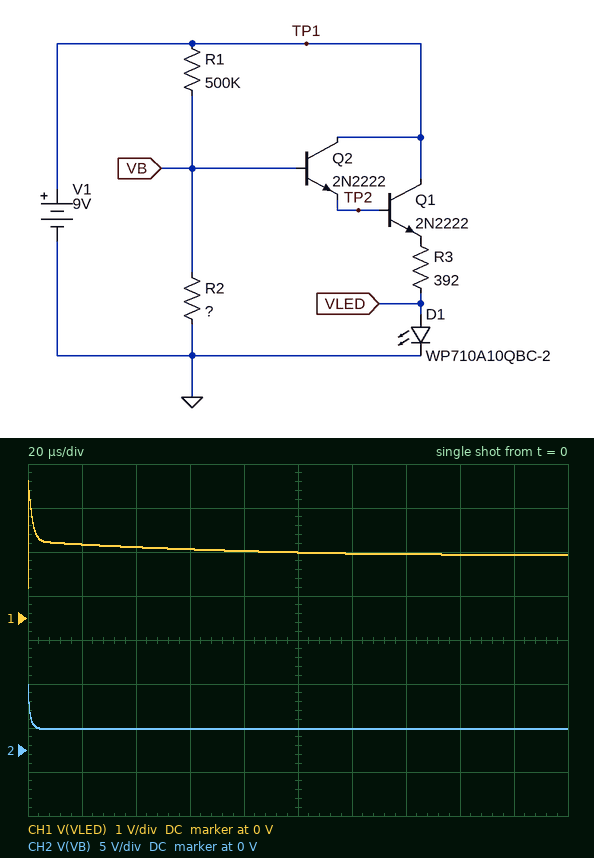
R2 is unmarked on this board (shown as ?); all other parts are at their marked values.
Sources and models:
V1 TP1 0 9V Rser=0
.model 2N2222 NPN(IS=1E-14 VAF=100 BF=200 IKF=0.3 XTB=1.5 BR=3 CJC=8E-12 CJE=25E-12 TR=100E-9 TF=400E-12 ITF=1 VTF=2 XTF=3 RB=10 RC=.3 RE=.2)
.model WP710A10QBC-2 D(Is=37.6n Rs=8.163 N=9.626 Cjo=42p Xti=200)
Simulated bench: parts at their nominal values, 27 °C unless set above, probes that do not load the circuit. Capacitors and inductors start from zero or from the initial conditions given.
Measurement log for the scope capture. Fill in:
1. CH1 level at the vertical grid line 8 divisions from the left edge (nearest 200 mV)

1.4 V
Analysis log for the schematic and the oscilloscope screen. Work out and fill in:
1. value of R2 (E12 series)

180 kΩ
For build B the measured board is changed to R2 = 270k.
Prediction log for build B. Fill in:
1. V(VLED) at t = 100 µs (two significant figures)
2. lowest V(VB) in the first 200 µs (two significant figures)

2.0 V
3.1 V
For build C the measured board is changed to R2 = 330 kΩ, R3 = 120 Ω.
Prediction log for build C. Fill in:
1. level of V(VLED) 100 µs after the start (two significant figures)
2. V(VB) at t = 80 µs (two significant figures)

2.4 V
3.6 V
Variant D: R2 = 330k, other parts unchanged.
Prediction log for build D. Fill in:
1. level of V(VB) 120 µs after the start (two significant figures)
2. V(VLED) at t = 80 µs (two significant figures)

3.6 V
2.3 V
